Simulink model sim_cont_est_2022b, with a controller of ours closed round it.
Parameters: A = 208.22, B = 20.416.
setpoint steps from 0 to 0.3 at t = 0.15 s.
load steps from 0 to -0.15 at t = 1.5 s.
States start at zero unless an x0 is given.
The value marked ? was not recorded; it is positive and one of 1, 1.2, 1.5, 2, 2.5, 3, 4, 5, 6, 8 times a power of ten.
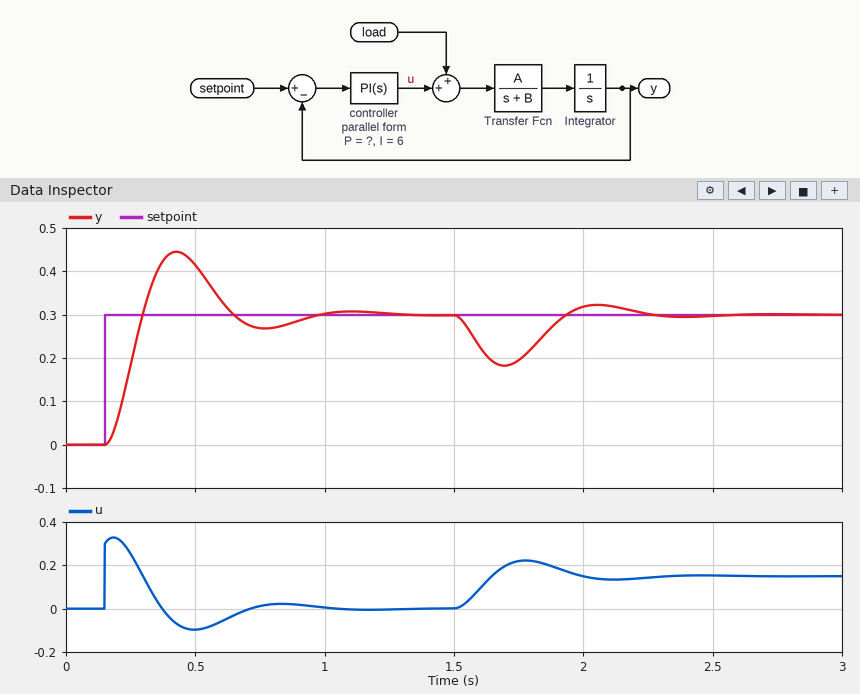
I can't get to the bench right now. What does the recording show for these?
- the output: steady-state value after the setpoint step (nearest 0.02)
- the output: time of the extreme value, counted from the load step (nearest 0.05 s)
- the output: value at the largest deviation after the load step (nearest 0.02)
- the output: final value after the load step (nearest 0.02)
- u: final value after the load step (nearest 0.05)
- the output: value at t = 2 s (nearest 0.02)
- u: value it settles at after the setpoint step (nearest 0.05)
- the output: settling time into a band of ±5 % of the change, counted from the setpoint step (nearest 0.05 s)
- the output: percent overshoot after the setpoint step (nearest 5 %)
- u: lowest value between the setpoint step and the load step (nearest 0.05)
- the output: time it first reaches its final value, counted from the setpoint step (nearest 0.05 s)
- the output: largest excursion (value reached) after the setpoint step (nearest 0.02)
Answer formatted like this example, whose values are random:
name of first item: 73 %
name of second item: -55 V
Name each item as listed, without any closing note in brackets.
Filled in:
the output: steady-state value after the setpoint step: 0.30
the output: time of the extreme value, counted from the load step: 0.20 s
the output: value at the largest deviation after the load step: 0.18
the output: final value after the load step: 0.30
u: final value after the load step: 0.15
the output: value at t = 2 s: 0.32
u: value it settles at after the setpoint step: 0.00
the output: settling time into a band of ±5 % of the change, counted from the setpoint step: 0.75 s
the output: percent overshoot after the setpoint step: 50 %
u: lowest value between the setpoint step and the load step: -0.10
the output: time it first reaches its final value, counted from the setpoint step: 0.15 s
the output: largest excursion (value reached) after the setpoint step: 0.44
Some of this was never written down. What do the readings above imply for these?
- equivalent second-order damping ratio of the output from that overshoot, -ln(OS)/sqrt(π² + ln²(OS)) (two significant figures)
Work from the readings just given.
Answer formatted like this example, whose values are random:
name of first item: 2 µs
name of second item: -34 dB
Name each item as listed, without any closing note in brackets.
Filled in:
equivalent second-order damping ratio of the output from that overshoot, -ln(OS)/sqrt(π² + ln²(OS)): 0.22
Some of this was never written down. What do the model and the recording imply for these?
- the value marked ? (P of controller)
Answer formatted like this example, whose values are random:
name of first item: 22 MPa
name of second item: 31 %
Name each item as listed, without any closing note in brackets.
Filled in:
the value marked ?: 1
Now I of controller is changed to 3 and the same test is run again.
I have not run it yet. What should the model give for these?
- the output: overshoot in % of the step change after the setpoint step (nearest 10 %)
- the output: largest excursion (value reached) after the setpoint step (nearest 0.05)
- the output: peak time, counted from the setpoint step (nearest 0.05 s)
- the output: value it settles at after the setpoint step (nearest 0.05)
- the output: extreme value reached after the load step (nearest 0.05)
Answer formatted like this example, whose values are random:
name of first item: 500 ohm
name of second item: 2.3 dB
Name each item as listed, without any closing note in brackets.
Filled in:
the output: overshoot in % of the step change after the setpoint step: 30 %
the output: largest excursion (value reached) after the setpoint step: 0.40
the output: peak time, counted from the setpoint step: 0.30 s
the output: value it settles at after the setpoint step: 0.30
the output: extreme value reached after the load step: 0.15
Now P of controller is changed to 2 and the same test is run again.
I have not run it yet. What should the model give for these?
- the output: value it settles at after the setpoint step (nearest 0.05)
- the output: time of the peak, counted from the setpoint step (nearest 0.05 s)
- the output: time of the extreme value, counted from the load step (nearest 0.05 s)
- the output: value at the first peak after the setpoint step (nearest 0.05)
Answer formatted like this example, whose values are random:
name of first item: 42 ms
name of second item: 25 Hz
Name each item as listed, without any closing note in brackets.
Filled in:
the output: value it settles at after the setpoint step: 0.30
the output: time of the peak, counted from the setpoint step: 0.20 s
the output: time of the extreme value, counted from the load step: 0.15 s
the output: value at the first peak after the setpoint step: 0.40
